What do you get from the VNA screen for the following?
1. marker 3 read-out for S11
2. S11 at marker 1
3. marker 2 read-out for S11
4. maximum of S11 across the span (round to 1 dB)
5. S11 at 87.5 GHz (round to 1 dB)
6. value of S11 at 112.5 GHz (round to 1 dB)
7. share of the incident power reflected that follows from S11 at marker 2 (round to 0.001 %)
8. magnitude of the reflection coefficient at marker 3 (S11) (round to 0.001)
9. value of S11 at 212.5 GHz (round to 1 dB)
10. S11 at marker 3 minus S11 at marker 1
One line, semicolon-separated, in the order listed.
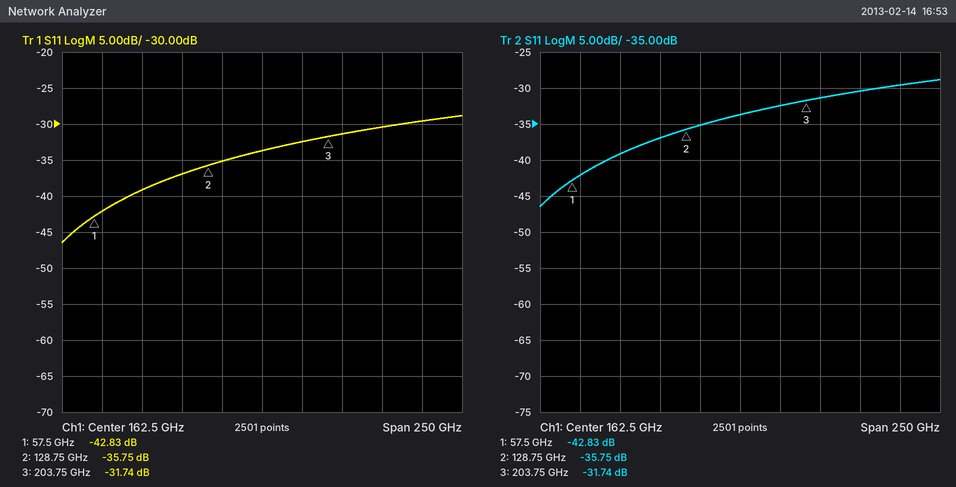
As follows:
-31.74 dB; -42.83 dB; -35.75 dB; -29 dB; -39 dB; -37 dB; 0.027 %; 0.026; -31 dB; 11.09 dB
